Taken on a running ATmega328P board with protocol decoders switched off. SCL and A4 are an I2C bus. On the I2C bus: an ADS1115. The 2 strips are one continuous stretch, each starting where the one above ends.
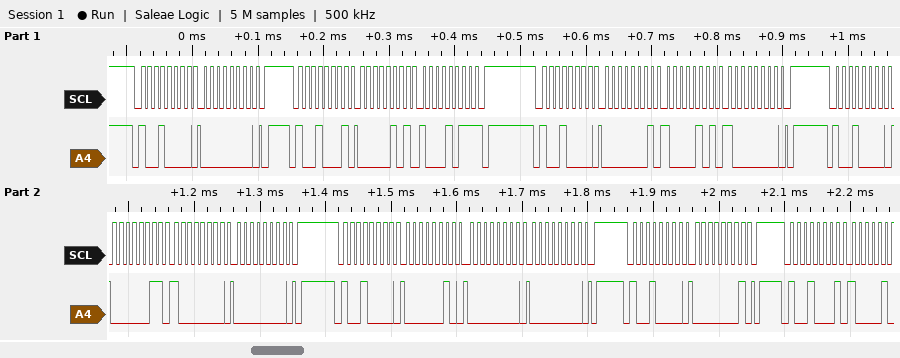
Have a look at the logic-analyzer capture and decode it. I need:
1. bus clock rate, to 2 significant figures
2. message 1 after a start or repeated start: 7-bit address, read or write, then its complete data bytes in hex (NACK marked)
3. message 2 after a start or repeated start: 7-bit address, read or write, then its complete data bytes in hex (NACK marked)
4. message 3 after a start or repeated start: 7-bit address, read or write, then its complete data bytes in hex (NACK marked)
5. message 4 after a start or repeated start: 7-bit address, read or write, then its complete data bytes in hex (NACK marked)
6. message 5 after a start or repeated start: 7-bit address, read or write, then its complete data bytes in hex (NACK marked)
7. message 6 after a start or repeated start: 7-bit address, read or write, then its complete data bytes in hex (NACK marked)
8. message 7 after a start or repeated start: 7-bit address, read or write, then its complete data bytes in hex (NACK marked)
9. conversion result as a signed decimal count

100 kHz
0x48 write: 00
0x48 read: 05 8B NACK
0x48 write: 01 85 80
0x48 write: 03 80 00
0x48 write: 02 00 00
0x48 write: 01
0x48 read
1419
